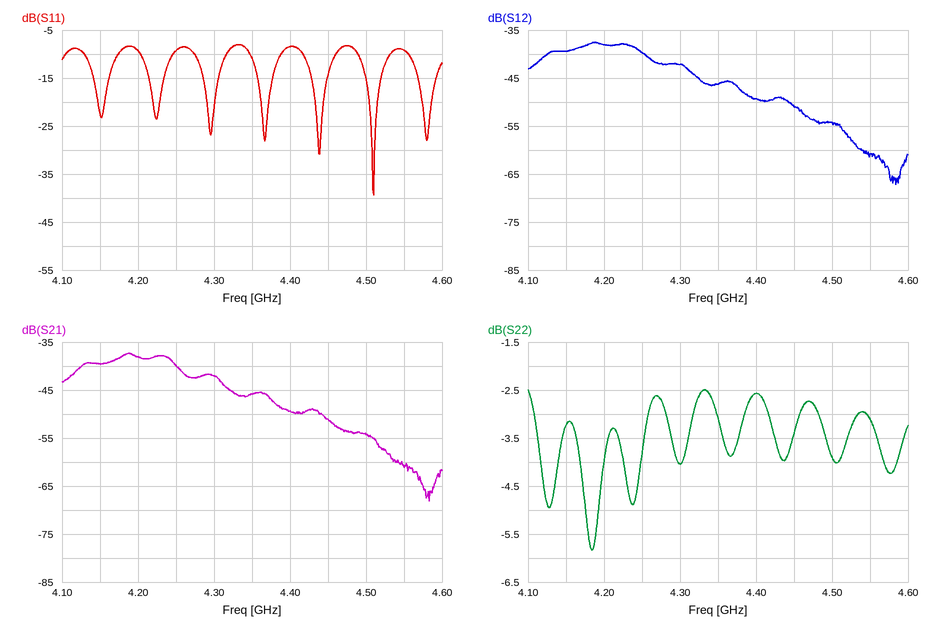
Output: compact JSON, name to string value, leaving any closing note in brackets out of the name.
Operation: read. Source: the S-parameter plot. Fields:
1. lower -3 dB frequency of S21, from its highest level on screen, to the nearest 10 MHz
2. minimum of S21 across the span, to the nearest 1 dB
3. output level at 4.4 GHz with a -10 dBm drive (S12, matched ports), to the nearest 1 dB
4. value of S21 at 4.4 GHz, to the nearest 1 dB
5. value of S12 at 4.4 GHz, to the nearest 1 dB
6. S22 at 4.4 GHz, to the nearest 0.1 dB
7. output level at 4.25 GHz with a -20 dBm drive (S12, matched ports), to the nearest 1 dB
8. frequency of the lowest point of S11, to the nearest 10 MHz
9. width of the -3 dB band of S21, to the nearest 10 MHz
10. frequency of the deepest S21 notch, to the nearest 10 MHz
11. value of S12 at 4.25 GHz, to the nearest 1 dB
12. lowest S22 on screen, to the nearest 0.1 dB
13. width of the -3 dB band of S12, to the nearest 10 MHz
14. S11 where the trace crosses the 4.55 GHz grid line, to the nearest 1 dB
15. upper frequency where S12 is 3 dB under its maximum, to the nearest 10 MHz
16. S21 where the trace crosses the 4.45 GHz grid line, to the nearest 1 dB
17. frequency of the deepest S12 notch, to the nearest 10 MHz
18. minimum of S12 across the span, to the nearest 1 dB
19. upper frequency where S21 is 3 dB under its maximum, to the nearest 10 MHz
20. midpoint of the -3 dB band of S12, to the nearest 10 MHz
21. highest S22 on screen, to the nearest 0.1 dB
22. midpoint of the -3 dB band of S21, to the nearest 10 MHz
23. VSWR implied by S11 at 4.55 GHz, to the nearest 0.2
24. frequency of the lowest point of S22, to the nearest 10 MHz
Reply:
{"lower -3 dB frequency of S21, from its highest level on screen, to the nearest 10 MHz": "4.12 GHz", "minimum of S21 across the span, to the nearest 1 dB": "-68 dB", "output level at 4.4 GHz with a -10 dBm drive (S12, matched ports), to the nearest 1 dB": "-59 dBm", "value of S21 at 4.4 GHz, to the nearest 1 dB": "-49 dB", "value of S12 at 4.4 GHz, to the nearest 1 dB": "-49 dB", "S22 at 4.4 GHz, to the nearest 0.1 dB": "-2.6 dB", "output level at 4.25 GHz with a -20 dBm drive (S12, matched ports), to the nearest 1 dB": "-60 dBm", "frequency of the lowest point of S11, to the nearest 10 MHz": "4.51 GHz", "width of the -3 dB band of S21, to the nearest 10 MHz": "130 MHz", "frequency of the deepest S21 notch, to the nearest 10 MHz": "4.58 GHz", "value of S12 at 4.25 GHz, to the nearest 1 dB": "-40 dB", "lowest S22 on screen, to the nearest 0.1 dB": "-5.8 dB", "width of the -3 dB band of S12, to the nearest 10 MHz": "140 MHz", "S11 where the trace crosses the 4.55 GHz grid line, to the nearest 1 dB": "-9 dB", "upper frequency where S12 is 3 dB under its maximum, to the nearest 10 MHz": "4.26 GHz", "S21 where the trace crosses the 4.45 GHz grid line, to the nearest 1 dB": "-51 dB", "frequency of the deepest S12 notch, to the nearest 10 MHz": "4.58 GHz", "minimum of S12 across the span, to the nearest 1 dB": "-67 dB", "upper frequency where S21 is 3 dB under its maximum, to the nearest 10 MHz": "4.25 GHz", "midpoint of the -3 dB band of S12, to the nearest 10 MHz": "4.19 GHz", "highest S22 on screen, to the nearest 0.1 dB": "-2.5 dB", "midpoint of the -3 dB band of S21, to the nearest 10 MHz": "4.19 GHz", "VSWR implied by S11 at 4.55 GHz, to the nearest 0.2": "2.0", "frequency of the lowest point of S22, to the nearest 10 MHz": "4.18 GHz"}
